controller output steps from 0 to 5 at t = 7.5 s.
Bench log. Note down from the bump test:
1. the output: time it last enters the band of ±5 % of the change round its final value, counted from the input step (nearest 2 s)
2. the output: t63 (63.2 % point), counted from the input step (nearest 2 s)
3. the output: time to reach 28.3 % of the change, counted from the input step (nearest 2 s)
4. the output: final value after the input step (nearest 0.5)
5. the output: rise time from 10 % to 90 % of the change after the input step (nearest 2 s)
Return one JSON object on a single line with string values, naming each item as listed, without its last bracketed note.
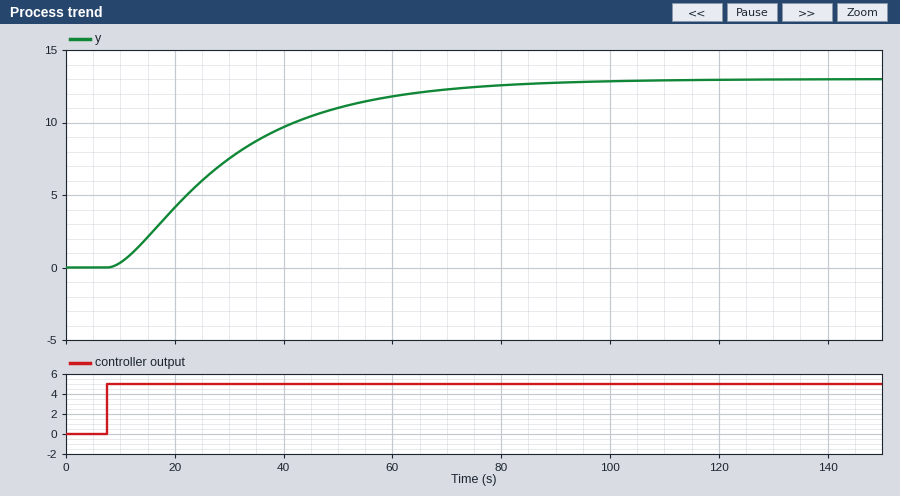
{"the output: time it last enters the band of ±5 % of the change round its final value, counted from the input step": "64 s", "the output: t63 (63.2 % point), counted from the input step": "26 s", "the output: time to reach 28.3 % of the change, counted from the input step": "12 s", "the output: final value after the input step": "13.0", "the output: rise time from 10 % to 90 % of the change after the input step": "46 s"}
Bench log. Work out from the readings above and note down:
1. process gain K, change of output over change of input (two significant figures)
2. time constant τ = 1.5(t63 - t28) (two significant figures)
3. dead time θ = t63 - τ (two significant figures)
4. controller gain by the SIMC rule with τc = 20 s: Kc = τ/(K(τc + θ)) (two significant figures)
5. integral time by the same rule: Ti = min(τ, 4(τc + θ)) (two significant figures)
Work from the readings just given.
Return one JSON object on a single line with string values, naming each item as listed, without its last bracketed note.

{"process gain K, change of output over change of input": "2.6", "time constant τ = 1.5(t63 - t28)": "21 s", "dead time θ = t63 - τ": "5.0 s", "controller gain by the SIMC rule with τc = 20 s: Kc = τ/(K(τc + θ))": "0.32", "integral time by the same rule: Ti = min(τ, 4(τc + θ))": "21 s"}
